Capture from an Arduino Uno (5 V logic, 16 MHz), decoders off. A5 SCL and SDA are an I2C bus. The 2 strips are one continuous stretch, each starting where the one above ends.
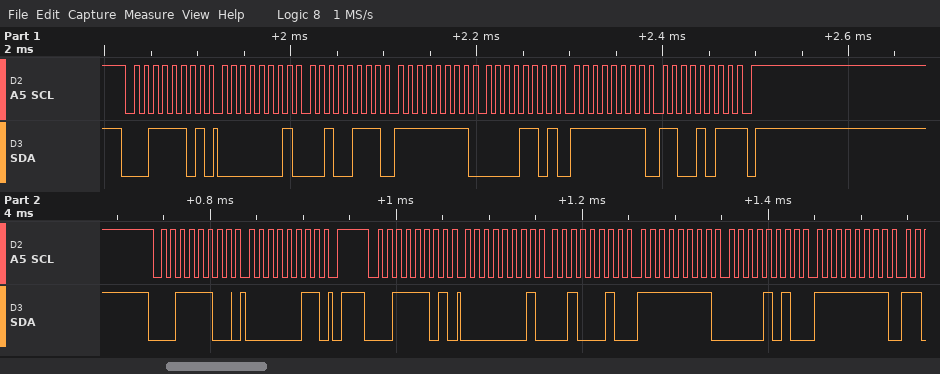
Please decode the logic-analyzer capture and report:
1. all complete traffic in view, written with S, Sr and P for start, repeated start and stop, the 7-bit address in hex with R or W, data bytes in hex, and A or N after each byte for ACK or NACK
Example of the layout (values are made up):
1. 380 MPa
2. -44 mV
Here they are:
1. S 1ER A 01 A 27 A FF A 0D A FF A CB N P S 1EW A 03 A P S 1ER A 01 A 22 A FF A 0A A FF A
